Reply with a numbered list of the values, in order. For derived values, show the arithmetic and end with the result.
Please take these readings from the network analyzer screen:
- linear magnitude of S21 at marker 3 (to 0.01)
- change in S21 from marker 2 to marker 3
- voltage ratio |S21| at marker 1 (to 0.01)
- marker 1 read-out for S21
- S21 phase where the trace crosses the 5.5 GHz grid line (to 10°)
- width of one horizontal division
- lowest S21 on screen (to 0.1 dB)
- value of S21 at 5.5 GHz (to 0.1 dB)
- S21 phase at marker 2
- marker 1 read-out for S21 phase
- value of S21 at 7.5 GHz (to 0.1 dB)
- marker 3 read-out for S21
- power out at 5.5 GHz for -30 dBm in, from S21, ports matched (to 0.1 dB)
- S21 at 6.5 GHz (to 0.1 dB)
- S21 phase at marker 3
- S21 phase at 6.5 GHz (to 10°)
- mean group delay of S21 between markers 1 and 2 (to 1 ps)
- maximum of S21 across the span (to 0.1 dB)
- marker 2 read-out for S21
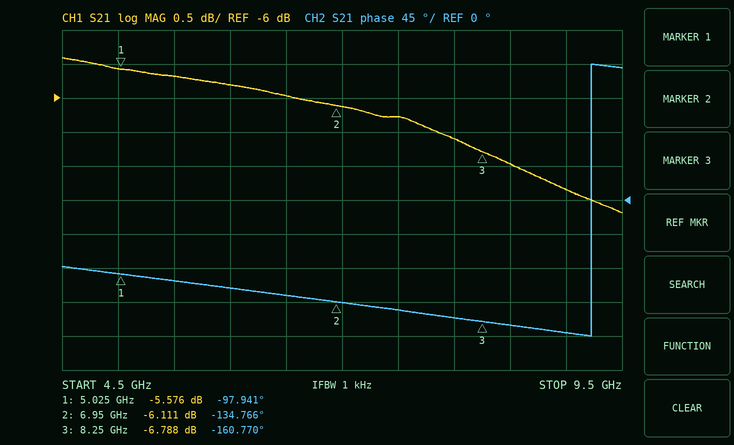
1. 10^(-6.788/20) ≈ 0.46
2. -6.788 − (-6.111) = -0.677 dB
3. 10^(-5.576/20) ≈ 0.53
4. -5.576 dB
5. -110°
6. 500 MHz
7. -7.7 dB
8. -5.7 dB
9. -134.766°
10. -97.941°
11. -6.3 dB
12. -6.788 dB
13. -30 dBm + (-5.7 dB) = -35.7 dBm
14. -6.0 dB
15. -160.770°
16. -130°
17. −(-134.766° − (-97.941°))/(360° × 1.925 GHz) ≈ 53 ps
18. -5.4 dB
19. -6.111 dB
